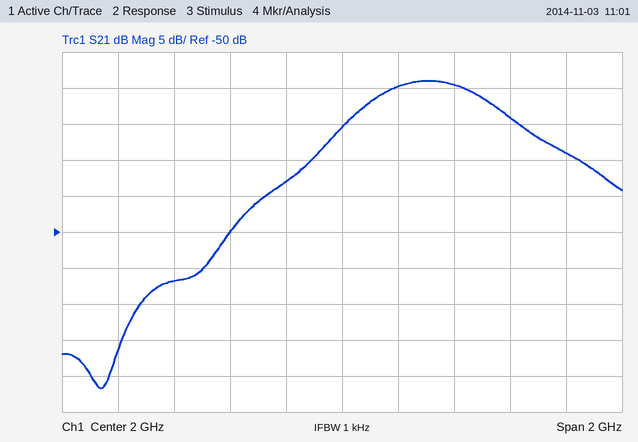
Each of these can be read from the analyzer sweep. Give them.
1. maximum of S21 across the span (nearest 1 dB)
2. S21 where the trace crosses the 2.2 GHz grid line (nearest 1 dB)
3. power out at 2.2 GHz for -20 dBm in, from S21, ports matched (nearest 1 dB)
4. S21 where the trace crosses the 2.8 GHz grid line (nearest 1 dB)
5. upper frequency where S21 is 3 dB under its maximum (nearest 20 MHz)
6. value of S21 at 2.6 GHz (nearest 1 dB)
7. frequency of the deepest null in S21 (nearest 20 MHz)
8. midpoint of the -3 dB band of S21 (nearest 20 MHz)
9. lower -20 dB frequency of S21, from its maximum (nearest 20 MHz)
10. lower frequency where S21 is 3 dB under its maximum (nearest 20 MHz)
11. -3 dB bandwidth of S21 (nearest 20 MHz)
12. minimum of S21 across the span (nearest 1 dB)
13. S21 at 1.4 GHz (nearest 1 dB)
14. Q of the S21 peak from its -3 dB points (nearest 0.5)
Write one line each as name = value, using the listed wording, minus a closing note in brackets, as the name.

maximum of S21 across the span = -29 dB
S21 where the trace crosses the 2.2 GHz grid line = -30 dB
power out at 2.2 GHz for -20 dBm in, from S21, ports matched = -50 dBm
S21 where the trace crosses the 2.8 GHz grid line = -39 dB
upper frequency where S21 is 3 dB under its maximum = 2.52 GHz
value of S21 at 2.6 GHz = -34 dB
frequency of the deepest null in S21 = 1.14 GHz
midpoint of the -3 dB band of S21 = 2.32 GHz
lower -20 dB frequency of S21, from its maximum = 1.62 GHz
lower frequency where S21 is 3 dB under its maximum = 2.10 GHz
-3 dB bandwidth of S21 = 420 MHz
minimum of S21 across the span = -72 dB
S21 at 1.4 GHz = -57 dB
Q of the S21 peak from its -3 dB points = 5.5
